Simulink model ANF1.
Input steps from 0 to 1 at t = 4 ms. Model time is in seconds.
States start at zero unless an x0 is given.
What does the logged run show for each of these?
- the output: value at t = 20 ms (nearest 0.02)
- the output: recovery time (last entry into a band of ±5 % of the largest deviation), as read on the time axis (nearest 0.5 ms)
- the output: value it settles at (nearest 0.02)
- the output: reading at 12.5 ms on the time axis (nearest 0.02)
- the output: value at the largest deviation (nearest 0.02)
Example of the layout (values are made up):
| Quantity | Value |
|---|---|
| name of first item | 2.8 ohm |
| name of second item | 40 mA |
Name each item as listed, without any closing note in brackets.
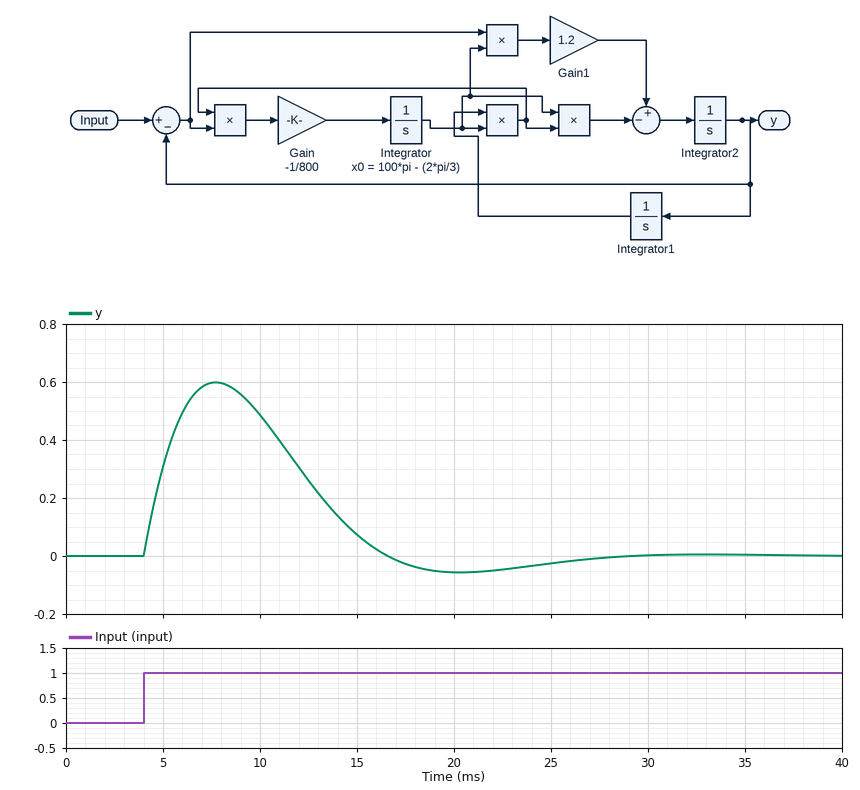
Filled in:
| Quantity | Value |
|---|---|
| the output: value at t = 20 ms | -0.06 |
| the output: recovery time (last entry into a band of ±5 % of the largest deviation), as read on the time axis | 24.5 ms |
| the output: value it settles at | 0.00 |
| the output: reading at 12.5 ms on the time axis | 0.26 |
| the output: value at the largest deviation | 0.60 |
